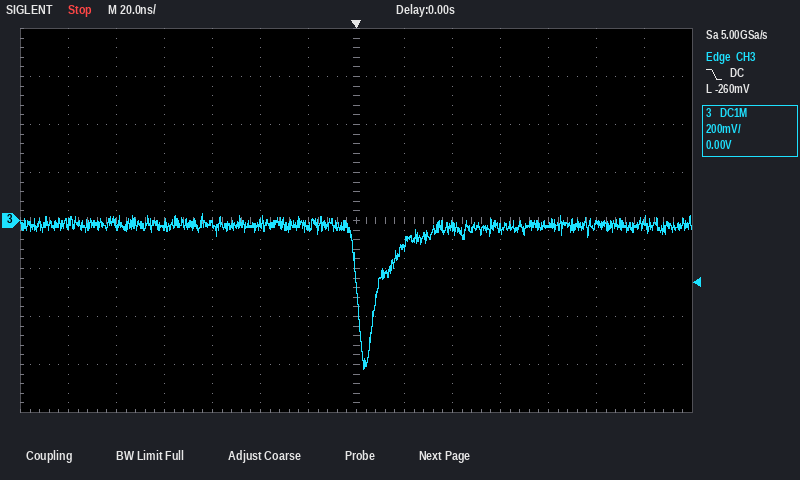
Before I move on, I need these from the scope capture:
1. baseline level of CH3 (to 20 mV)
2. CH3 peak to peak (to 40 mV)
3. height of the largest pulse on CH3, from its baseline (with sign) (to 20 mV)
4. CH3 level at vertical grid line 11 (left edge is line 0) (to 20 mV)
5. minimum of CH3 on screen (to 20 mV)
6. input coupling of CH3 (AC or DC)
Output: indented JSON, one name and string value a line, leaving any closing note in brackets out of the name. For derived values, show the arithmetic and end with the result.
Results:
{
  "baseline level of CH3": "-20 mV",
  "CH3 peak to peak": "640 mV",
  "height of the largest pulse on CH3, from its baseline (with sign)": "-620 mV − (-20 mV) = -600 mV",
  "CH3 level at vertical grid line 11 (left edge is line 0)": "-20 mV",
  "minimum of CH3 on screen": "-620 mV",
  "input coupling of CH3": "DC"
}
